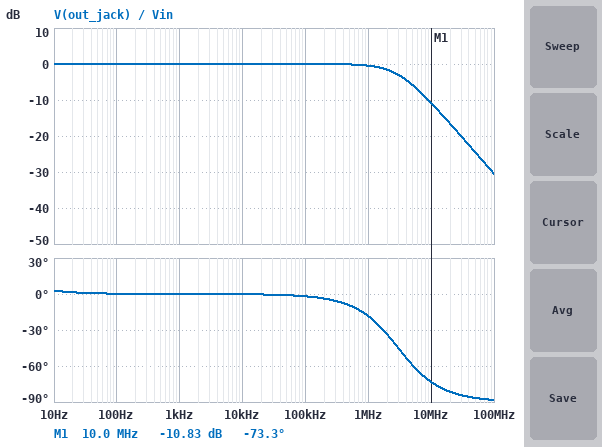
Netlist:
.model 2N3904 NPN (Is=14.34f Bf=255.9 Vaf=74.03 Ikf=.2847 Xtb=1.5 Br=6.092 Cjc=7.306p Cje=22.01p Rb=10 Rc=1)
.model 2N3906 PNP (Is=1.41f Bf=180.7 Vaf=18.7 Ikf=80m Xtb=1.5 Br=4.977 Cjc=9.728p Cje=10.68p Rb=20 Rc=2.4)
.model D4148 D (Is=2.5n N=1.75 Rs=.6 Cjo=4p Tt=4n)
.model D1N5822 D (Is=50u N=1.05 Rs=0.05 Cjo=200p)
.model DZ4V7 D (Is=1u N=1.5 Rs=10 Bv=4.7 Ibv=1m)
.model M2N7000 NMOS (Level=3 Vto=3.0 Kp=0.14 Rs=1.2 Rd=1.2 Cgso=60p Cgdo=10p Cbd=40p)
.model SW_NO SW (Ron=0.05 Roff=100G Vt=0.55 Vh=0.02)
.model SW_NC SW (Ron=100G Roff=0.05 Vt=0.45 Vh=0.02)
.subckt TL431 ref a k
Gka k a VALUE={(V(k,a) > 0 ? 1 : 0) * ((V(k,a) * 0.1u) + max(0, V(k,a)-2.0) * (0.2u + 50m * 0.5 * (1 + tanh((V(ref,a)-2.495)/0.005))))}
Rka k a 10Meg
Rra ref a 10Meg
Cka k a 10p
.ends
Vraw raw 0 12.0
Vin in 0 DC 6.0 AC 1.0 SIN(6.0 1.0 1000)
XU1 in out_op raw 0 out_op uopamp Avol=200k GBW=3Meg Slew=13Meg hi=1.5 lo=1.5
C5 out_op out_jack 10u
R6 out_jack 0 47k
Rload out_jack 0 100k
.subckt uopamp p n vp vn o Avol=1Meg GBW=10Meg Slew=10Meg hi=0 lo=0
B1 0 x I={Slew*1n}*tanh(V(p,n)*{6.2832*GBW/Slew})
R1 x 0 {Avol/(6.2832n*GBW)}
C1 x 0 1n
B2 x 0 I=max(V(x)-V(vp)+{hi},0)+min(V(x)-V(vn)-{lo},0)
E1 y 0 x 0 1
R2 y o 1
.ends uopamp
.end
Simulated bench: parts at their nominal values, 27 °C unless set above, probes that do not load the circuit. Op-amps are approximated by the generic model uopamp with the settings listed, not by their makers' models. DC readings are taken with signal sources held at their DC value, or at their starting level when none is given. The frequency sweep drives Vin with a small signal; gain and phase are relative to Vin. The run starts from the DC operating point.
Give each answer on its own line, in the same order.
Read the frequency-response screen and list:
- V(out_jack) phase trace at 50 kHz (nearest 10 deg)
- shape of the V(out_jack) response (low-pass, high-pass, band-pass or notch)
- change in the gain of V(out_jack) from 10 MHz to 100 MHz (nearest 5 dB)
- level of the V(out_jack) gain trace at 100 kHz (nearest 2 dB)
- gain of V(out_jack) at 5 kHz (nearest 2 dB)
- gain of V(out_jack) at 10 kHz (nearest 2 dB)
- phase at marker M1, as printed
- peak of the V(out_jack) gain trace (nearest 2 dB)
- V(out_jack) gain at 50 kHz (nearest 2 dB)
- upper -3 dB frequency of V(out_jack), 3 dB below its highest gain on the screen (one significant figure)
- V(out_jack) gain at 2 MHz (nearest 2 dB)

0 deg
low-pass
-20 dB
0 dB
0 dB
0 dB
-73.3 deg
0 dB
0 dB
3 MHz
-2 dB
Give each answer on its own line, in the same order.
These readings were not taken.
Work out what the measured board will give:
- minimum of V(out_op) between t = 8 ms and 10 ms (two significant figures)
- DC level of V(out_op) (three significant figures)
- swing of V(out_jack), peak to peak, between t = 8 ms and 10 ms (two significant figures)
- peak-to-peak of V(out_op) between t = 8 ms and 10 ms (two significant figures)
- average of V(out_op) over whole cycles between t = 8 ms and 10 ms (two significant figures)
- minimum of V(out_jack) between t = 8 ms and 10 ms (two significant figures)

5.0 V
6.00 V
2.0 V
2.0 V
6.0 V
-1.0 V
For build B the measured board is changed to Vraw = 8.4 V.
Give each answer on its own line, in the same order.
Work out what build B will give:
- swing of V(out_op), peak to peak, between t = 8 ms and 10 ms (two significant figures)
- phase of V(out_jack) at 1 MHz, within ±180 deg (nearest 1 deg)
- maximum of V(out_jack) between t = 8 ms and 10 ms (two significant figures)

1.9 V
-18 deg
900 mV
